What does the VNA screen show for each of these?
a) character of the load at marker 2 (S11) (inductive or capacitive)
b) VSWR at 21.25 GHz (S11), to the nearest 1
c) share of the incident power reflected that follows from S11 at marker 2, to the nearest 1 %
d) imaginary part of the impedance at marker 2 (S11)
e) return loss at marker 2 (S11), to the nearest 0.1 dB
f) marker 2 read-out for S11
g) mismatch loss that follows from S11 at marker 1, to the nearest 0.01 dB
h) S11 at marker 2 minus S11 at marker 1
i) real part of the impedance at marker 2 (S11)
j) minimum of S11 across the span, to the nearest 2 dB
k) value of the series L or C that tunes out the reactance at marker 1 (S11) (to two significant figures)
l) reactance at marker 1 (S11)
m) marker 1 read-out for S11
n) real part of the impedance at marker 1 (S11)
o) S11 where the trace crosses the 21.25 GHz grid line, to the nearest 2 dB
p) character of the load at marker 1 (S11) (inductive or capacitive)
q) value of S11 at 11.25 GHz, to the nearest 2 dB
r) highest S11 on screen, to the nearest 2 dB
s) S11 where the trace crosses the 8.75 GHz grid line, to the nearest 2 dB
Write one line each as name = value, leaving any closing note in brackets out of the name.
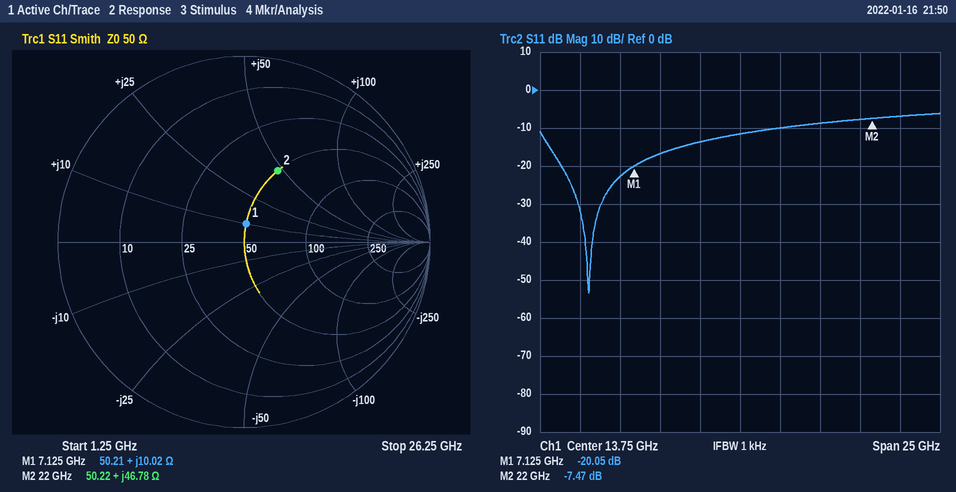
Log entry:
character of the load at marker 2 (S11) = inductive
VSWR at 21.25 GHz (S11), to the nearest 1 = 2
share of the incident power reflected that follows from S11 at marker 2, to the nearest 1 % = 18 %
imaginary part of the impedance at marker 2 = +46.78 Ω
return loss at marker 2 (S11), to the nearest 0.1 dB = 7.5 dB
marker 2 read-out for S11 = -7.47 dB
mismatch loss that follows from S11 at marker 1, to the nearest 0.01 dB = 0.04 dB
S11 at marker 2 minus S11 at marker 1 = 12.58 dB
real part of the impedance at marker 2 = 50.22 Ω
minimum of S11 across the span, to the nearest 2 dB = -54 dB
value of the series L or C that tunes out the reactance at marker 1 (S11) = 2.2 pF
reactance at marker 1 = +10.02 Ω
marker 1 read-out for S11 = -20.05 dB
real part of the impedance at marker 1 = 50.21 Ω
S11 where the trace crosses the 21.25 GHz grid line, to the nearest 2 dB = -8 dB
character of the load at marker 1 (S11) = inductive
value of S11 at 11.25 GHz, to the nearest 2 dB = -14 dB
highest S11 on screen, to the nearest 2 dB = -6 dB
S11 where the trace crosses the 8.75 GHz grid line, to the nearest 2 dB = -16 dB
